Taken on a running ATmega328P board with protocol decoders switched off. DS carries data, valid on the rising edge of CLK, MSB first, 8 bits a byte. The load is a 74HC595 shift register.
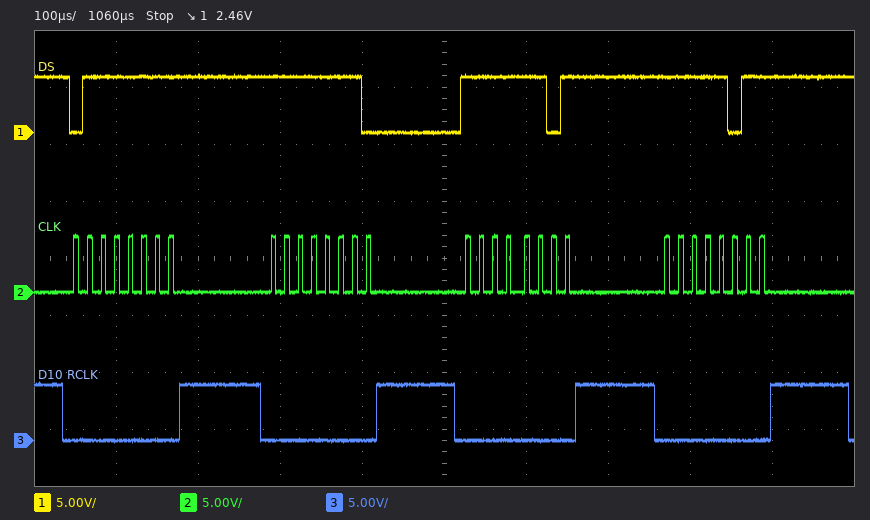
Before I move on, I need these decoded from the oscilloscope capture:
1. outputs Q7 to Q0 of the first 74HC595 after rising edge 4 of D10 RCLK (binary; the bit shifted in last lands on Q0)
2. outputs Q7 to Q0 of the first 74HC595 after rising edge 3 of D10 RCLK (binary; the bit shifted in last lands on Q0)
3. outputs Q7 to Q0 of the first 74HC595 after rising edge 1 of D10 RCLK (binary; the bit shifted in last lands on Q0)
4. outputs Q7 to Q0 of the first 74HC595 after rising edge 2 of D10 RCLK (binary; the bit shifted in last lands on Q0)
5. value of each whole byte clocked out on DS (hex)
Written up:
11111011
11111101
01111111
11111110
7F FE FD FB
